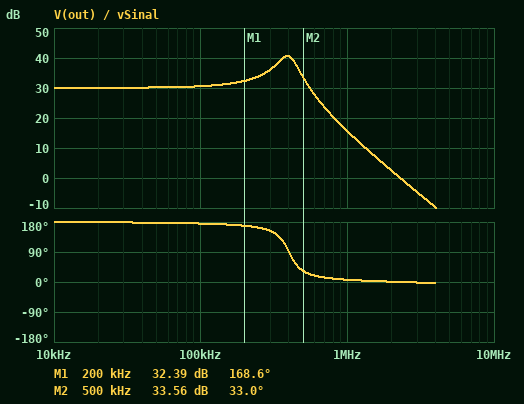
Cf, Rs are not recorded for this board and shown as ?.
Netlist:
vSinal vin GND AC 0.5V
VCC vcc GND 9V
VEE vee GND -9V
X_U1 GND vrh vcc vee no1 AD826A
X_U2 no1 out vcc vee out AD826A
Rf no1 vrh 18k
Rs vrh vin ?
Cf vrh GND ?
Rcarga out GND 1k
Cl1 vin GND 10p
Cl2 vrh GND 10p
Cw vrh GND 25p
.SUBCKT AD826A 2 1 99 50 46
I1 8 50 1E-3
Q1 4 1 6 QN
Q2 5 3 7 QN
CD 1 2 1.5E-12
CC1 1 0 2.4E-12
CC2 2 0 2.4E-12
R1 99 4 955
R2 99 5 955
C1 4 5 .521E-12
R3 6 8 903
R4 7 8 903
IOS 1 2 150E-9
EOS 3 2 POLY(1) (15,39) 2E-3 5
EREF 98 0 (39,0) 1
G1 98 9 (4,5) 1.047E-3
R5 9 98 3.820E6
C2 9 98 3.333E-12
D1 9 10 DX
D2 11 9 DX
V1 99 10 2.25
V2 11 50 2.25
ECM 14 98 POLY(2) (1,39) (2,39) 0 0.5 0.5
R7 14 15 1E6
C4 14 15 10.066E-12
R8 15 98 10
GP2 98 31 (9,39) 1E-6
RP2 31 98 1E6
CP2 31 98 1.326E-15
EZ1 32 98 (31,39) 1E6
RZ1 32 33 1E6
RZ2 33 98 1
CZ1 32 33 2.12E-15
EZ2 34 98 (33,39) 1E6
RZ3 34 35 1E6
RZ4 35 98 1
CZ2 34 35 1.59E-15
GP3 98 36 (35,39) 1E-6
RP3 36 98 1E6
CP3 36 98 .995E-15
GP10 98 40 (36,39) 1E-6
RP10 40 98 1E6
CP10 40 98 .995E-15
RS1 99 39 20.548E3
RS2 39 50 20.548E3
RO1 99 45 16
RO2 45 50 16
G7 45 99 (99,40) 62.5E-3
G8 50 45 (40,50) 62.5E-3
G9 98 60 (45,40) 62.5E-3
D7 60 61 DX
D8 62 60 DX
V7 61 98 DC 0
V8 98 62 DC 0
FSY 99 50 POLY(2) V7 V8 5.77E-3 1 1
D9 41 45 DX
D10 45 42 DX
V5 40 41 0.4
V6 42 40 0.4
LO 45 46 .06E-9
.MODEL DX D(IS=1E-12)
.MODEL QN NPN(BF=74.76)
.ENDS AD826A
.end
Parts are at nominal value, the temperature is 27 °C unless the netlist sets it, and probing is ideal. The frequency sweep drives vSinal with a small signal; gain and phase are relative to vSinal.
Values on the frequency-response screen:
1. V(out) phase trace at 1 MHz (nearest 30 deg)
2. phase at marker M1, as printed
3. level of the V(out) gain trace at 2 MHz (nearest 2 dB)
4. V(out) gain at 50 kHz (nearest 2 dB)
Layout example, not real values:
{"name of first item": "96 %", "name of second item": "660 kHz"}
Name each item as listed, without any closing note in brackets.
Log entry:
{"V(out) phase trace at 1 MHz": "0 deg", "phase at marker M1, as printed": "168.6 deg", "level of the V(out) gain trace at 2 MHz": "2 dB", "V(out) gain at 50 kHz": "30 dB"}
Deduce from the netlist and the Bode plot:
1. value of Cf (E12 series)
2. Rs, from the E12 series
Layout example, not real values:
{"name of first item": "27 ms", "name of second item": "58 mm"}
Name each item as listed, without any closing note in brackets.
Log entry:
{"value of Cf": "2.7 nF", "Rs, from the E12 series": "560 Ω"}
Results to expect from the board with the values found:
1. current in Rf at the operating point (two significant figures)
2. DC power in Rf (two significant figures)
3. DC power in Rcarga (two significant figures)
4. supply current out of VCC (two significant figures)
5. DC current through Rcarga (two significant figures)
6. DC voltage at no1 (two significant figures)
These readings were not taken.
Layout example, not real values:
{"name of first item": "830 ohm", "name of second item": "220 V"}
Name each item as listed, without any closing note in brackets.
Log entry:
{"current in Rf at the operating point": "10 µA", "DC power in Rf": "1.9 µW", "DC power in Rcarga": "35 µW", "supply current out of VCC": "15 mA", "DC current through Rcarga": "190 µA", "DC voltage at no1": "190 mV"}
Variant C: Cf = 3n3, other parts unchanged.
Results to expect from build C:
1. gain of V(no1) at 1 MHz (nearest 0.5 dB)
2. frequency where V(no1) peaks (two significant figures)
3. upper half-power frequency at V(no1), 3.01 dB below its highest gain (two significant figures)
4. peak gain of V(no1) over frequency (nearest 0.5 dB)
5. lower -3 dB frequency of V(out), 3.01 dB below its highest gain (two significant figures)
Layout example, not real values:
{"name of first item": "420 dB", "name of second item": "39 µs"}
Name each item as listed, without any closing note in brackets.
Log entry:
{"gain of V(no1) at 1 MHz": "13.5 dB", "frequency where V(no1) peaks": "360 kHz", "upper half-power frequency at V(no1), 3.01 dB below its highest gain": "400 kHz", "peak gain of V(no1) over frequency": "41.5 dB", "lower -3 dB frequency of V(out), 3.01 dB below its highest gain": "300 kHz"}
